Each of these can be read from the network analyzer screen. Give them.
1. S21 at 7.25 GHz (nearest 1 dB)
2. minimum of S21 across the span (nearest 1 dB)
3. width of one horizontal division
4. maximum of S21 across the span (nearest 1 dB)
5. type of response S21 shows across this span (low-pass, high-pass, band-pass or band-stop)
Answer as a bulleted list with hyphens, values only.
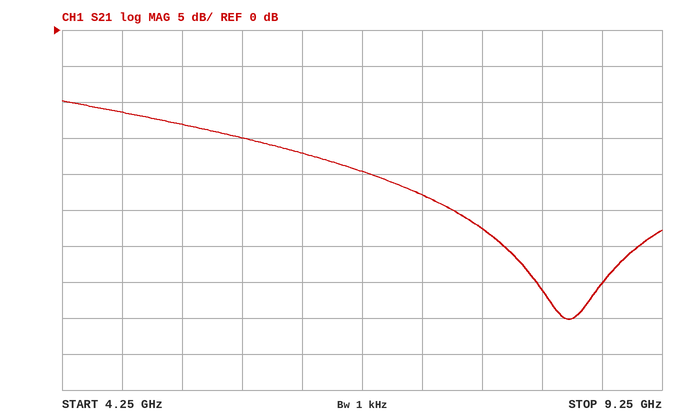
- -23 dB
- -40 dB
- 500 MHz
- -10 dB
- low-pass
